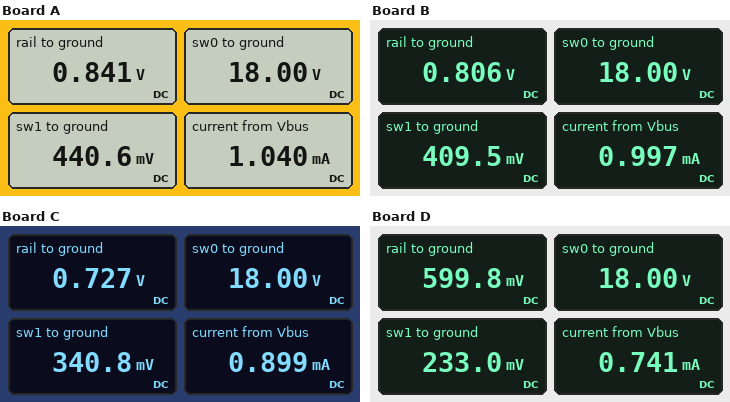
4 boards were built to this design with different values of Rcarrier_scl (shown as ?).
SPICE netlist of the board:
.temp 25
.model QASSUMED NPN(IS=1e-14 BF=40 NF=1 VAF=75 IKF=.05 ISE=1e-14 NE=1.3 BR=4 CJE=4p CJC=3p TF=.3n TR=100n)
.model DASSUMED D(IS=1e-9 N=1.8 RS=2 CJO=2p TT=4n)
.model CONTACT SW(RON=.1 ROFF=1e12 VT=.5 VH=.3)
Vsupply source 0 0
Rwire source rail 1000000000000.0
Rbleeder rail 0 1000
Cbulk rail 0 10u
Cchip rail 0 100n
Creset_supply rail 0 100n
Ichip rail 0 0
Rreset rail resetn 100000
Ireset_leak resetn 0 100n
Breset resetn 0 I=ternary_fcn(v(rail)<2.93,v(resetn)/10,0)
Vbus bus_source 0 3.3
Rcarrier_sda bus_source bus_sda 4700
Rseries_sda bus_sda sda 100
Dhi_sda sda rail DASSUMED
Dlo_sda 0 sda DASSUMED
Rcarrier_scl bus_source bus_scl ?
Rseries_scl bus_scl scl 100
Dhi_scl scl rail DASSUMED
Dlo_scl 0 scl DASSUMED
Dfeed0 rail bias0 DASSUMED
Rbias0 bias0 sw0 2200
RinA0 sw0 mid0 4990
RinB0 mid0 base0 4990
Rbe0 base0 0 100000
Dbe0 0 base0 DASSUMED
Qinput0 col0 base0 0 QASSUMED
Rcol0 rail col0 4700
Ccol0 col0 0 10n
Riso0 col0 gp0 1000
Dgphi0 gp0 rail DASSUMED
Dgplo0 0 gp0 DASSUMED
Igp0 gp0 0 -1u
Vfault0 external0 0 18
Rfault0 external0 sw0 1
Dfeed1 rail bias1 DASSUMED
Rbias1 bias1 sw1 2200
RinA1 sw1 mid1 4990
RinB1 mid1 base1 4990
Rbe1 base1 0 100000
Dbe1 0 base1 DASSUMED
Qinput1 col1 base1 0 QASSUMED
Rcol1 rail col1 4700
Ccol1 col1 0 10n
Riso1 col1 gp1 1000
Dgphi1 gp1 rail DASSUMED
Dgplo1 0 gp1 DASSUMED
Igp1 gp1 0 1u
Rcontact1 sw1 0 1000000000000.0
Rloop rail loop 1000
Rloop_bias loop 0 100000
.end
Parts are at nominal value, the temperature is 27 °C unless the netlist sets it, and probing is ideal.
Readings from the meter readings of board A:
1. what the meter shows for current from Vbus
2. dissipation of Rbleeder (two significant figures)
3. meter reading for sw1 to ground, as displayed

1.040 mA
710 µW
440.6 mV
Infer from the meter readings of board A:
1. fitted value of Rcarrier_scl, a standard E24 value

2.7 kΩ
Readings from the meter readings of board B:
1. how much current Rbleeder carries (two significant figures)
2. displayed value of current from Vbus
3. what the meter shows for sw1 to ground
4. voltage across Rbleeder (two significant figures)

810 µA
0.997 mA
409.5 mV
810 mV
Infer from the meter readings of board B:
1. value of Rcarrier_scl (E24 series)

3 kΩ
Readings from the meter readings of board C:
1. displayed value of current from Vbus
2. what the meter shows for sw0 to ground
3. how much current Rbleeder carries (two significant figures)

0.899 mA
18.00 V
730 µA
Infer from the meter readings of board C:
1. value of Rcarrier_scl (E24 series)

3.9 kΩ
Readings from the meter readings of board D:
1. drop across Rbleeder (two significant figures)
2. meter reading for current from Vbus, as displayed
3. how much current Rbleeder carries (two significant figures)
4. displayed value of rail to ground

600 mV
0.741 mA
600 µA
599.8 mV
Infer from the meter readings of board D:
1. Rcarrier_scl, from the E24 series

6.8 kΩ
